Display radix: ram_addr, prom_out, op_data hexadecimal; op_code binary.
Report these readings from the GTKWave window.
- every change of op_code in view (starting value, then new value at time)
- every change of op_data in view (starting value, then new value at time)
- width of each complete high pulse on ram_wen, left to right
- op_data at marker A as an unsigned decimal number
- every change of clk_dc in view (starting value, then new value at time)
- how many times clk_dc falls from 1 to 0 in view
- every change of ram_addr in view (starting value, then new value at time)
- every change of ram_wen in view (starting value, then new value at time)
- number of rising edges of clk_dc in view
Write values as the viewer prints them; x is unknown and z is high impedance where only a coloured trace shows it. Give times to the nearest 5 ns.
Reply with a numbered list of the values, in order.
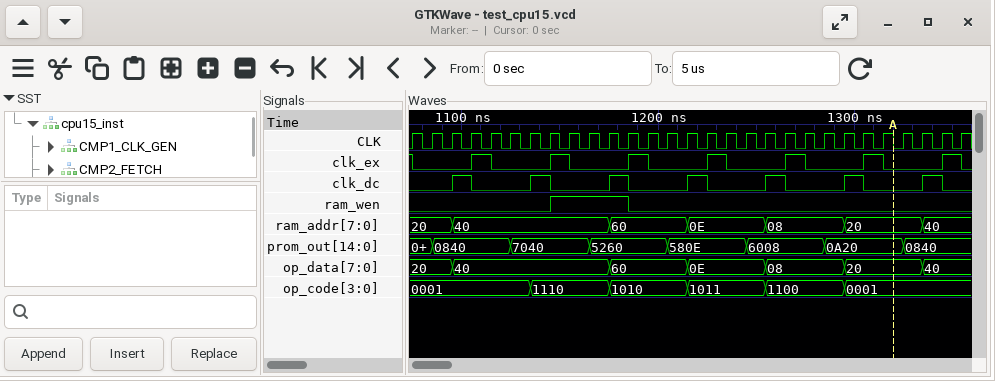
1. 0001, 1110 at 1135 ns, 1010 at 1175 ns, 1011 at 1215 ns, 1100 at 1255 ns, 0001 at 1295 ns
2. 20, 40 at 1095 ns, 60 at 1175 ns, 0E at 1215 ns, 08 at 1255 ns, 20 at 1295 ns, 40 at 1335 ns
3. 40 ns
4. 32
5. 0, 1 at 1095 ns, 0 at 1105 ns, 1 at 1135 ns, 0 at 1145 ns, 1 at 1175 ns, 0 at 1185 ns, 1 at 1215 ns, 0 at 1225 ns, 1 at 1255 ns, 0 at 1265 ns, 1 at 1295 ns, 0 at 1305 ns, 1 at 1335 ns, 0 at 1345 ns
6. 7
7. 20, 40 at 1095 ns, 60 at 1175 ns, 0E at 1215 ns, 08 at 1255 ns, 20 at 1295 ns, 40 at 1335 ns
8. 0, 1 at 1145 ns, 0 at 1185 ns
9. 7
